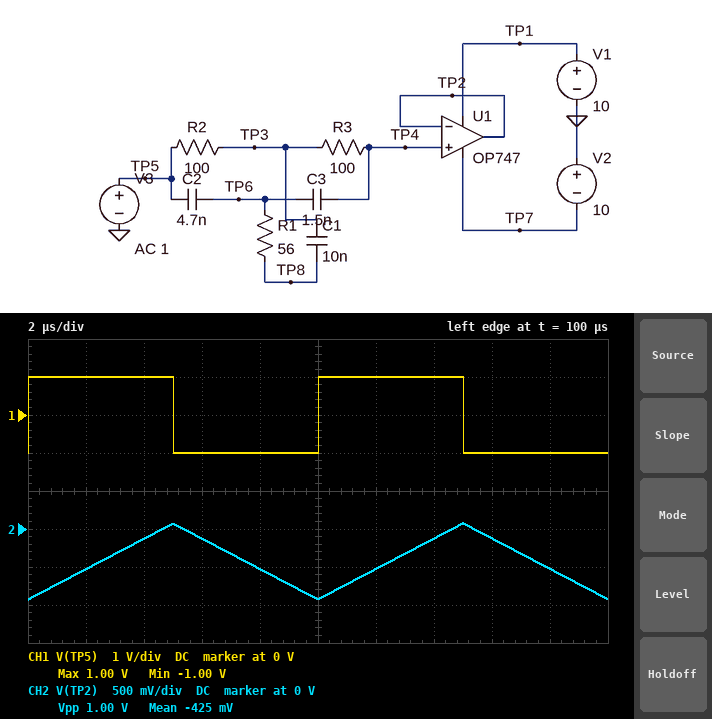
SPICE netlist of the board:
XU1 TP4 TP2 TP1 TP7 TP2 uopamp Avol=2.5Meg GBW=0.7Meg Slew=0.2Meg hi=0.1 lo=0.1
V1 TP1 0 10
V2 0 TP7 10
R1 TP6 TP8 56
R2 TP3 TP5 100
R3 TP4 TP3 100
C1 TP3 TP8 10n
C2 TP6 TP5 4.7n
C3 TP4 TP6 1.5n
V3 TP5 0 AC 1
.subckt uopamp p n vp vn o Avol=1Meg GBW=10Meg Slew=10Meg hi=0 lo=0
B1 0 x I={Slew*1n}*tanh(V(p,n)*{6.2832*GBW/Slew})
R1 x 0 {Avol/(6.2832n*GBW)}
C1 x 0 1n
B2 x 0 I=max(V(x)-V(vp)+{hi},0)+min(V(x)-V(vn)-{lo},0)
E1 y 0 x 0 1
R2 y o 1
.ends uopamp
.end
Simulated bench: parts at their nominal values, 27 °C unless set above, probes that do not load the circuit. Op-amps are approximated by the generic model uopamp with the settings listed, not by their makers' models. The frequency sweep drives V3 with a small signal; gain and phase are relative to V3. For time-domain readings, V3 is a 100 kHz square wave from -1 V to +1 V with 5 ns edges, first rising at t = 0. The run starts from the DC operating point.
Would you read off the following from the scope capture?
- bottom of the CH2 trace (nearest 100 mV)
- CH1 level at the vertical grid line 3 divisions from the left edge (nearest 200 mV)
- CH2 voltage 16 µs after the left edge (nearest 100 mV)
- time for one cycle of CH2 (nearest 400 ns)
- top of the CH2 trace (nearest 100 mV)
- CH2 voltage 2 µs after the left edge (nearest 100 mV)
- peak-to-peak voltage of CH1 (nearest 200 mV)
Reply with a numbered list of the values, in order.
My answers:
1. -900 mV
2. -1.0 V
3. -100 mV
4. 10.0 µs
5. 100 mV
6. -500 mV
7. 2.0 V
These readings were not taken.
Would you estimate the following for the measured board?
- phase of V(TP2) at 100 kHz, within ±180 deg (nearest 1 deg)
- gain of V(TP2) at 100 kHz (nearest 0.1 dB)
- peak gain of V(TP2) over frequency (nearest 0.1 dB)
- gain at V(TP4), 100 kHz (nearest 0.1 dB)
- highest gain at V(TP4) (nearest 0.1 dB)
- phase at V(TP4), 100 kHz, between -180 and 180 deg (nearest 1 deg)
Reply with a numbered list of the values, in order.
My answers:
1. -8 deg
2. -0.1 dB
3. 0 dB
4. 0 dB
5. 0 dB
6. 0 deg
